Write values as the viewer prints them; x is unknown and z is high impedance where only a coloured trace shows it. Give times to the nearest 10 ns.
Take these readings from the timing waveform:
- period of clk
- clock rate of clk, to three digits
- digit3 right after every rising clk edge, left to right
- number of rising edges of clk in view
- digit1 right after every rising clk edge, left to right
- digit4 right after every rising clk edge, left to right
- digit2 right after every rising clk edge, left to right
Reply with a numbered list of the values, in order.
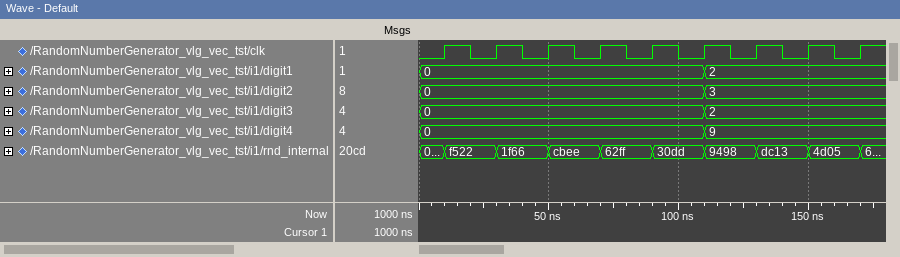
1. 20 ns
2. 50.0 MHz
3. 0, 0, 0, 0, 0, 2, 2, 2, 2
4. 9
5. 0, 0, 0, 0, 0, 2, 2, 2, 2
6. 0, 0, 0, 0, 0, 9, 9, 9, 9
7. 0, 0, 0, 0, 0, 3, 3, 3, 3
